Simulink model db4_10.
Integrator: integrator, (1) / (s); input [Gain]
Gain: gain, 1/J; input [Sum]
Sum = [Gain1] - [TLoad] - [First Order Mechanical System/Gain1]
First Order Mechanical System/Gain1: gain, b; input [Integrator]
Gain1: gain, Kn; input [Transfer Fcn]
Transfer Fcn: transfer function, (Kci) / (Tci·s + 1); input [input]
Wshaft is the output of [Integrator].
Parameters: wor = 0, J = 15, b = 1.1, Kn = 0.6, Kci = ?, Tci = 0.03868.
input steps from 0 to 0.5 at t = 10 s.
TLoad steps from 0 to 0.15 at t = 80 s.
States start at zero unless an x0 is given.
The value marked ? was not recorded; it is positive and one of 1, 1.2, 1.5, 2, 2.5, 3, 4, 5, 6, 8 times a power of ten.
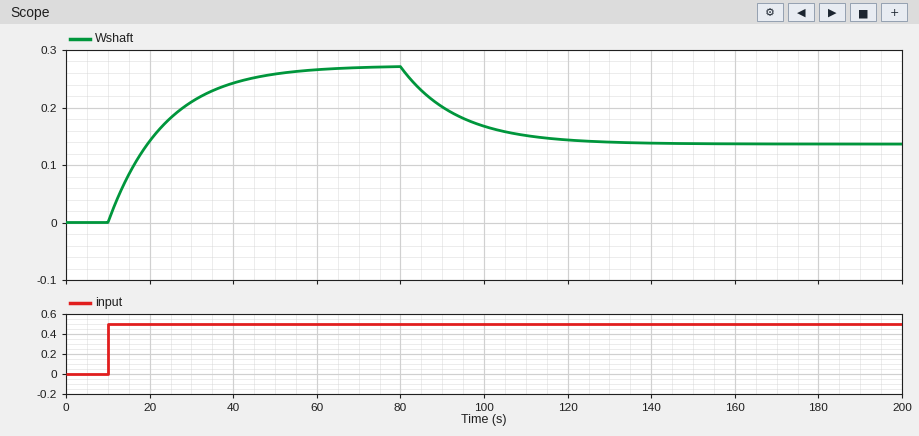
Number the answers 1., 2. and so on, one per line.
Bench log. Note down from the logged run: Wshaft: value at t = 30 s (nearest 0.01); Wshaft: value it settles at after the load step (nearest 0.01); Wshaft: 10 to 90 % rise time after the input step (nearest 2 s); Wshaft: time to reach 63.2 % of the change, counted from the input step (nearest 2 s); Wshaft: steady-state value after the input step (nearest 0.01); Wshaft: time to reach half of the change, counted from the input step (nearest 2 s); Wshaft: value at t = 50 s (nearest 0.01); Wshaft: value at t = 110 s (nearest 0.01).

1. 0.21
2. 0.14
3. 30 s
4. 14 s
5. 0.27
6. 10 s
7. 0.26
8. 0.15
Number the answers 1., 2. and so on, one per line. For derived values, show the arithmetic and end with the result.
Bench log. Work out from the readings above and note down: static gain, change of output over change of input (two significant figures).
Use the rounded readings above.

1. (0.27 - 0) / (0.5 - 0) = 0.54
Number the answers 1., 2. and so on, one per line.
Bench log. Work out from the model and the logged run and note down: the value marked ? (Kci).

1. 1
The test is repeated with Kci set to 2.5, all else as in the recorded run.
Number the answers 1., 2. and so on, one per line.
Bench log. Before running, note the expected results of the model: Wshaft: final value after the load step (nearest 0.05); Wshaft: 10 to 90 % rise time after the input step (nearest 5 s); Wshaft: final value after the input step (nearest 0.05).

1. 0.55
2. 30 s
3. 0.70
